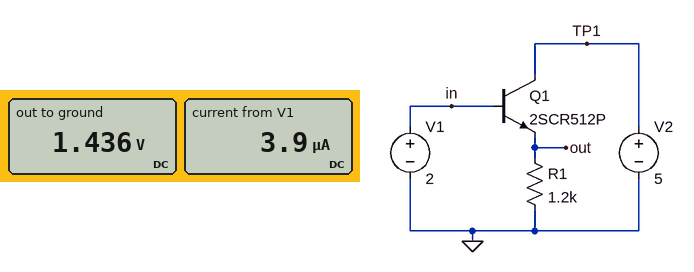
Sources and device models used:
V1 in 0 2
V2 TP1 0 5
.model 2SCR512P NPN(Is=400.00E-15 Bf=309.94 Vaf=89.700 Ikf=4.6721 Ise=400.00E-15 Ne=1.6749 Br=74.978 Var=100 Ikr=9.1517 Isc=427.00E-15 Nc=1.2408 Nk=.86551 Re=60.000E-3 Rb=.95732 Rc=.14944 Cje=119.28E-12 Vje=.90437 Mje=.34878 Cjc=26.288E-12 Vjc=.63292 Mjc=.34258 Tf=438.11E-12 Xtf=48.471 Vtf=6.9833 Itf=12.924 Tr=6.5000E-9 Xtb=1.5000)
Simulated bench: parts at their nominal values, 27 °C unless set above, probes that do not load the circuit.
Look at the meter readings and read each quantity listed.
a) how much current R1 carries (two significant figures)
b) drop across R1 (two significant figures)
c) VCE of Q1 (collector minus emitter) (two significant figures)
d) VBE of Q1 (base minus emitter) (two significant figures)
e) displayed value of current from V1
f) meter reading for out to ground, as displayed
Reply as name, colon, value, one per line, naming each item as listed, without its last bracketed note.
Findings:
how much current R1 carries: 1.2 mA
drop across R1: 1.4 V
VCE of Q1 (collector minus emitter): 3.6 V
VBE of Q1 (base minus emitter): 560 mV
displayed value of current from V1: 3.9 µA
meter reading for out to ground, as displayed: 1.436 V
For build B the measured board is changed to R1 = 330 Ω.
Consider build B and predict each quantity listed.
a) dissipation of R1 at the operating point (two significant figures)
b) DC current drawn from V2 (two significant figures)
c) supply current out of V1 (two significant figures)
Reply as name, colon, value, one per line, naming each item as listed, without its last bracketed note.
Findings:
dissipation of R1 at the operating point: 6.0 mW
DC current drawn from V2: 4.2 mA
supply current out of V1: 14 µA
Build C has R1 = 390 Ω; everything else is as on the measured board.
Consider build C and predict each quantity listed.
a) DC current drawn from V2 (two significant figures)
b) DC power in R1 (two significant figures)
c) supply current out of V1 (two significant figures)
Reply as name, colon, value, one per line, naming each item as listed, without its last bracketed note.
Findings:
DC current drawn from V2: 3.6 mA
DC power in R1: 5.1 mW
supply current out of V1: 12 µA
